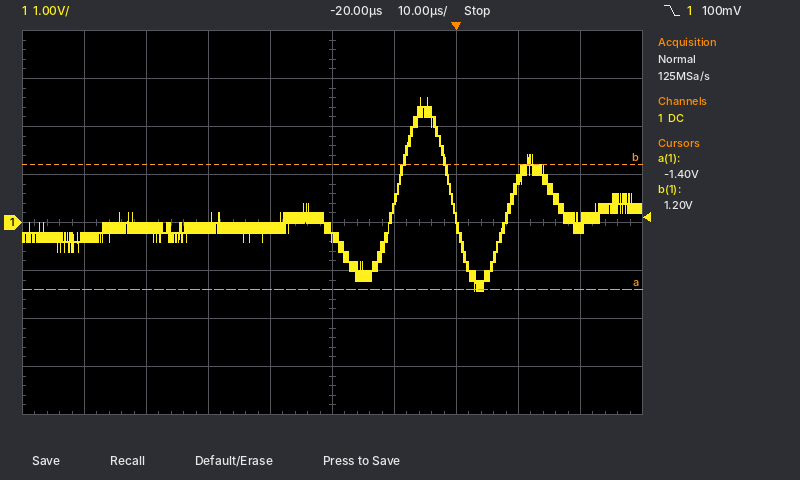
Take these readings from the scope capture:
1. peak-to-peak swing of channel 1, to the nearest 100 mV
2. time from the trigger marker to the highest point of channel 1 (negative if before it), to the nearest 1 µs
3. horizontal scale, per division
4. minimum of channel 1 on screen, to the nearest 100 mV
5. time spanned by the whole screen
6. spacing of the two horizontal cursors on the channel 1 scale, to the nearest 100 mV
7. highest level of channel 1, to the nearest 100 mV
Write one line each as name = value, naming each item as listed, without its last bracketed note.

peak-to-peak swing of channel 1, to the nearest 100 mV = 4.0 V
time from the trigger marker to the highest point of channel 1 (negative if before it), to the nearest 1 µs = -5 µs
horizontal scale, per division = 10 µs
minimum of channel 1 on screen, to the nearest 100 mV = -1.4 V
time spanned by the whole screen = 100 µs
spacing of the two horizontal cursors on the channel 1 scale, to the nearest 100 mV = 2.6 V
highest level of channel 1, to the nearest 100 mV = 2.6 V
